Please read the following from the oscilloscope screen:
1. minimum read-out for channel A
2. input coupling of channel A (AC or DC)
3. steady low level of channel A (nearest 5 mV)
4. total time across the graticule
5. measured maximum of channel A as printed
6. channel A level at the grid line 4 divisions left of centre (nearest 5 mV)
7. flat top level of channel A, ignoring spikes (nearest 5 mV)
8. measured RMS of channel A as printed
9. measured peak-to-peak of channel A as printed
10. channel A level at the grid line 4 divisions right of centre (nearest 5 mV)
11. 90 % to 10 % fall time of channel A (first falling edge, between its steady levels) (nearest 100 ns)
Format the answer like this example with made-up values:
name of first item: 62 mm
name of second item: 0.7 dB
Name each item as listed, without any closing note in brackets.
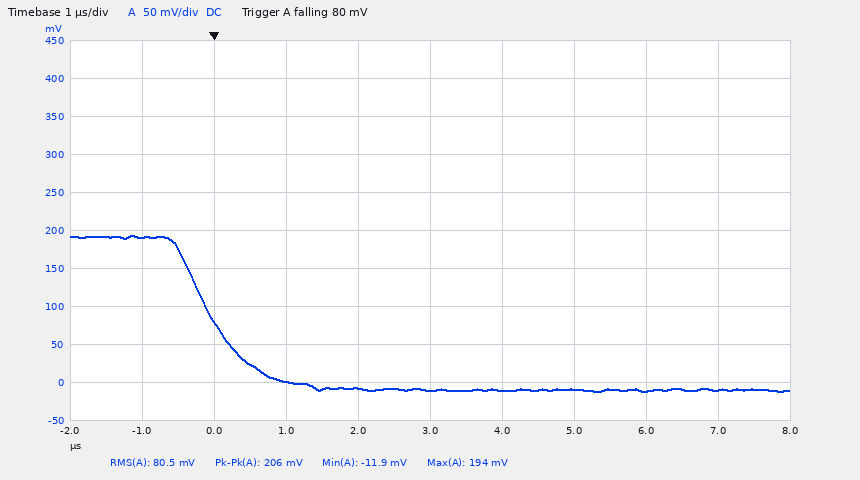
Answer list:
minimum read-out for channel A: -11.9 mV
input coupling of channel A: DC
steady low level of channel A: -10 mV
total time across the graticule: 10 µs
measured maximum of channel A as printed: 194 mV
channel A level at the grid line 4 divisions left of centre: 190 mV
flat top level of channel A, ignoring spikes: 190 mV
measured RMS of channel A as printed: 80.5 mV
measured peak-to-peak of channel A as printed: 206 mV
channel A level at the grid line 4 divisions right of centre: -10 mV
90 % to 10 % fall time of channel A (first falling edge, between its steady levels): 1.2 µs
